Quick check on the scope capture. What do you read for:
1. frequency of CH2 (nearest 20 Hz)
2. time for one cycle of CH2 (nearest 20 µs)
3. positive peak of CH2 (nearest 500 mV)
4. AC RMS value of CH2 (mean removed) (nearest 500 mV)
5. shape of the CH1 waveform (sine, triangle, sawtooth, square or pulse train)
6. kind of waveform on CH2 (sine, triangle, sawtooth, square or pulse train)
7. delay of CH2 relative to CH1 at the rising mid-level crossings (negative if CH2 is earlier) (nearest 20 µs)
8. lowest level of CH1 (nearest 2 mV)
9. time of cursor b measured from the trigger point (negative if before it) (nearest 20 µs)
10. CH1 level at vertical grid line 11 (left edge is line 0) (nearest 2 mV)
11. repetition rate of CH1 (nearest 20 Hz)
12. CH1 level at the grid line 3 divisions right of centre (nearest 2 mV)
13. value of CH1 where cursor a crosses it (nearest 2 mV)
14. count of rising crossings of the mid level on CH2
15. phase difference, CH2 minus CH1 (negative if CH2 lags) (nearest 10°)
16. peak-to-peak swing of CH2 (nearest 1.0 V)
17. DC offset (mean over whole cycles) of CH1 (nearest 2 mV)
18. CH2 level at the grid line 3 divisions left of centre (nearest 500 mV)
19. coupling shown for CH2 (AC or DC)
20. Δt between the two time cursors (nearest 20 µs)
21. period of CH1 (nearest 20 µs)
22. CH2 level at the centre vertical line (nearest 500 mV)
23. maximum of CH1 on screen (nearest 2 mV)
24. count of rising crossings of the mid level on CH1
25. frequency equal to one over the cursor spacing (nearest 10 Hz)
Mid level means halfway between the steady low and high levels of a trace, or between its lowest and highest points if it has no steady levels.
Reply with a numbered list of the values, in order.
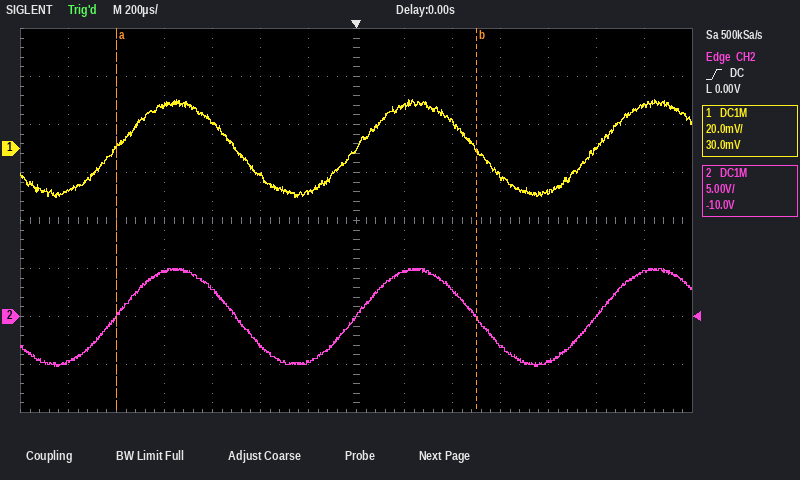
1. 1.00 kHz
2. 1.00 ms
3. 5.0 V
4. 3.5 V
5. sine
6. sine
7. 0 µs
8. -20 mV
9. +500 µs
10. -18 mV
11. 1.00 kHz
12. -12 mV
13. 0 mV
14. 3
15. 0°
16. 10.0 V
17. 0 mV
18. 3.0 V
19. DC
20. 1.50 ms
21. 1.00 ms
22. 0.0 V
23. 20 mV
24. 3
25. 670 Hz
